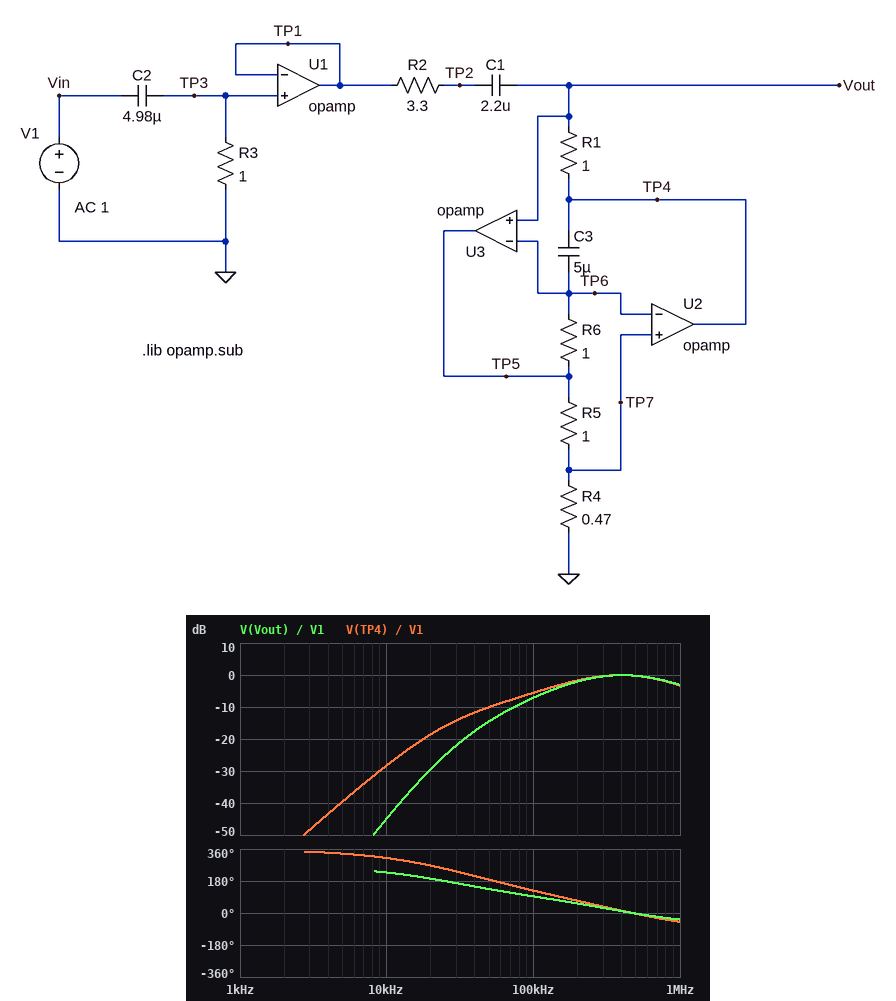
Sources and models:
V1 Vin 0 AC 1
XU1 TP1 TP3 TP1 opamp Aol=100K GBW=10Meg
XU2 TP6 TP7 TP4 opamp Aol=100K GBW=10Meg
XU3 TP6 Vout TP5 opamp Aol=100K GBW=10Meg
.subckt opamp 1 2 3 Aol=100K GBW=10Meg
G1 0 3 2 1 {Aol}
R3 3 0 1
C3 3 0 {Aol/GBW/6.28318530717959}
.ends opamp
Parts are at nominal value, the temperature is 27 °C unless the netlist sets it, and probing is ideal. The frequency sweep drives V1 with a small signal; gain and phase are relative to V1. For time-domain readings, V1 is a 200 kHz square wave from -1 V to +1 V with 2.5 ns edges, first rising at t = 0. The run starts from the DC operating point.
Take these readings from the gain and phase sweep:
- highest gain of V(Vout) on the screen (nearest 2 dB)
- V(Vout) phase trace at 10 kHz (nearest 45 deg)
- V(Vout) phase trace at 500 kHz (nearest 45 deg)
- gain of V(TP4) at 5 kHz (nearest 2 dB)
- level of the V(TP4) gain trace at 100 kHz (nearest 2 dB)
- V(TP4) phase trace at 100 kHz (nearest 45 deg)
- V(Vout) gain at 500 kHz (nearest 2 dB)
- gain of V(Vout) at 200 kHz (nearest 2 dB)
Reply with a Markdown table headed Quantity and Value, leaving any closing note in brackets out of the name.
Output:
| Quantity | Value |
|---|---|
| highest gain of V(Vout) on the screen | 0 dB |
| V(Vout) phase trace at 10 kHz | 225 deg |
| V(Vout) phase trace at 500 kHz | 0 deg |
| gain of V(TP4) at 5 kHz | -40 dB |
| level of the V(TP4) gain trace at 100 kHz | -6 dB |
| V(TP4) phase trace at 100 kHz | 135 deg |
| V(Vout) gain at 500 kHz | 0 dB |
| gain of V(Vout) at 200 kHz | -2 dB |
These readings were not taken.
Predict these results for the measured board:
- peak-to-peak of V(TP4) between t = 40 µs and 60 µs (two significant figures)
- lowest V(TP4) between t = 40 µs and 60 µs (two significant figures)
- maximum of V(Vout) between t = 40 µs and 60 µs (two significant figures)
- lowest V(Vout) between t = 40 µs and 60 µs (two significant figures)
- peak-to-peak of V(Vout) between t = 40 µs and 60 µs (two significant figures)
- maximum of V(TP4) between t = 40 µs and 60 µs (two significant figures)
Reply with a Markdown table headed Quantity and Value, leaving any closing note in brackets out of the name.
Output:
| Quantity | Value |
|---|---|
| peak-to-peak of V(TP4) between t = 40 µs and 60 µs | 3.3 V |
| lowest V(TP4) between t = 40 µs and 60 µs | -1.6 V |
| maximum of V(Vout) between t = 40 µs and 60 µs | 1.5 V |
| lowest V(Vout) between t = 40 µs and 60 µs | -1.5 V |
| peak-to-peak of V(Vout) between t = 40 µs and 60 µs | 3.1 V |
| maximum of V(TP4) between t = 40 µs and 60 µs | 1.6 V |
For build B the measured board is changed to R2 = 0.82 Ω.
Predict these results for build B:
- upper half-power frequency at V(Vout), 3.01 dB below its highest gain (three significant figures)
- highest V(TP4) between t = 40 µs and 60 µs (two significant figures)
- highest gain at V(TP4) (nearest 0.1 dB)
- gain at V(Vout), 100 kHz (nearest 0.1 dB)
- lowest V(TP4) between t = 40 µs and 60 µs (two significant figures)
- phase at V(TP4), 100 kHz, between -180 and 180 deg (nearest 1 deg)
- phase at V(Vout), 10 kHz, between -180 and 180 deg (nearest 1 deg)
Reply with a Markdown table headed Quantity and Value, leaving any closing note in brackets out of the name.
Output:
| Quantity | Value |
|---|---|
| upper half-power frequency at V(Vout), 3.01 dB below its highest gain | 890 kHz |
| highest V(TP4) between t = 40 µs and 60 µs | 1.9 V |
| highest gain at V(TP4) | 4.7 dB |
| gain at V(Vout), 100 kHz | 2.2 dB |
| lowest V(TP4) between t = 40 µs and 60 µs | -1.9 V |
| phase at V(TP4), 100 kHz, between -180 and 180 deg | 94 deg |
| phase at V(Vout), 10 kHz, between -180 and 180 deg | -114 deg |
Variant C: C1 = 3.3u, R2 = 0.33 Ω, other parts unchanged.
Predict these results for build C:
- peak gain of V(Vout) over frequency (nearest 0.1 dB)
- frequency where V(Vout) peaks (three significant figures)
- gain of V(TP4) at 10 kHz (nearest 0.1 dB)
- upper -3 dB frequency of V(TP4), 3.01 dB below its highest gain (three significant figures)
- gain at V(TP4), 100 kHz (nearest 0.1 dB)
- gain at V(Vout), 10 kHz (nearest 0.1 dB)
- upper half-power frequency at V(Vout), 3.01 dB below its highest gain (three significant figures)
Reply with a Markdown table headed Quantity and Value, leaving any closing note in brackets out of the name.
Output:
| Quantity | Value |
|---|---|
| peak gain of V(Vout) over frequency | 7.5 dB |
| frequency where V(Vout) peaks | 59.2 kHz |
| gain of V(TP4) at 10 kHz | -23.8 dB |
| upper -3 dB frequency of V(TP4), 3.01 dB below its highest gain | 72.1 kHz |
| gain at V(TP4), 100 kHz | 4.0 dB |
| gain at V(Vout), 10 kHz | -40.4 dB |
| upper half-power frequency at V(Vout), 3.01 dB below its highest gain | 78.0 kHz |
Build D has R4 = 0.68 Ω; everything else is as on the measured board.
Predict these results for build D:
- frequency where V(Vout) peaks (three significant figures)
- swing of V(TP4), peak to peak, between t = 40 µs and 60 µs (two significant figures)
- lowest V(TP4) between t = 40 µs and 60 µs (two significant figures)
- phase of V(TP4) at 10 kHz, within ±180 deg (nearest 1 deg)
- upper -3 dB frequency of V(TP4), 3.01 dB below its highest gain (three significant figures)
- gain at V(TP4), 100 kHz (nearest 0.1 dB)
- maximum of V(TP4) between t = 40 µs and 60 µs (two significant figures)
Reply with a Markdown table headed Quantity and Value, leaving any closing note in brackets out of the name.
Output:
| Quantity | Value |
|---|---|
| frequency where V(Vout) peaks | 375 kHz |
| swing of V(TP4), peak to peak, between t = 40 µs and 60 µs | 3.5 V |
| lowest V(TP4) between t = 40 µs and 60 µs | -1.7 V |
| phase of V(TP4) at 10 kHz, within ±180 deg | -55 deg |
| upper -3 dB frequency of V(TP4), 3.01 dB below its highest gain | 1.15 MHz |
| gain at V(TP4), 100 kHz | -3.7 dB |
| maximum of V(TP4) between t = 40 µs and 60 µs | 1.7 V |
